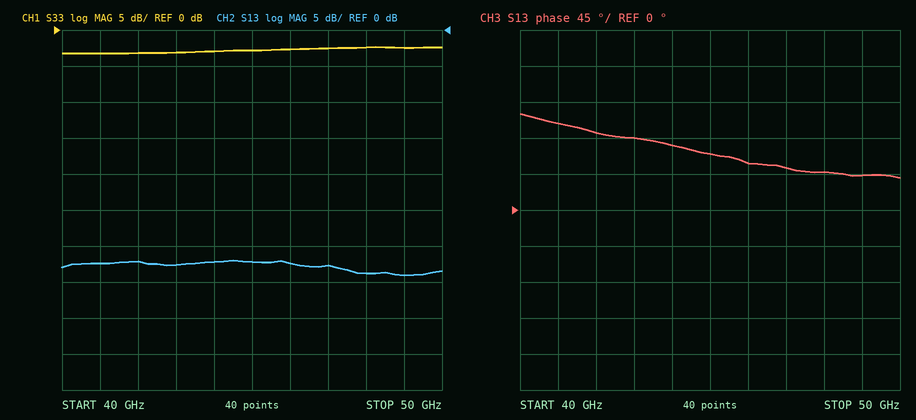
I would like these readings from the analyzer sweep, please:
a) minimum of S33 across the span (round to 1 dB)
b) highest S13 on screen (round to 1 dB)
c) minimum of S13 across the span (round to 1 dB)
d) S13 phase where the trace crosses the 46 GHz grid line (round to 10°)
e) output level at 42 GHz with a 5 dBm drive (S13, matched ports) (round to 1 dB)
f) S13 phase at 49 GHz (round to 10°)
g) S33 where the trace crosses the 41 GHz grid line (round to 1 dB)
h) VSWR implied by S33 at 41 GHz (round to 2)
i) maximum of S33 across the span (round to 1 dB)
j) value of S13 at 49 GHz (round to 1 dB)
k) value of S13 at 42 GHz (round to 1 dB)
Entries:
-3 dB
-32 dB
-34 dB
60°
-27 dBm
40°
-3 dB
6
-2 dB
-34 dB
-32 dB
